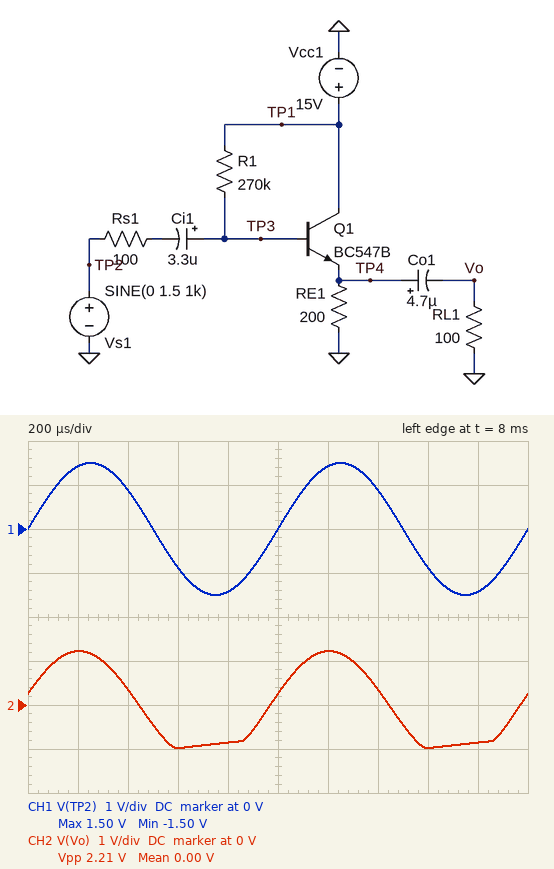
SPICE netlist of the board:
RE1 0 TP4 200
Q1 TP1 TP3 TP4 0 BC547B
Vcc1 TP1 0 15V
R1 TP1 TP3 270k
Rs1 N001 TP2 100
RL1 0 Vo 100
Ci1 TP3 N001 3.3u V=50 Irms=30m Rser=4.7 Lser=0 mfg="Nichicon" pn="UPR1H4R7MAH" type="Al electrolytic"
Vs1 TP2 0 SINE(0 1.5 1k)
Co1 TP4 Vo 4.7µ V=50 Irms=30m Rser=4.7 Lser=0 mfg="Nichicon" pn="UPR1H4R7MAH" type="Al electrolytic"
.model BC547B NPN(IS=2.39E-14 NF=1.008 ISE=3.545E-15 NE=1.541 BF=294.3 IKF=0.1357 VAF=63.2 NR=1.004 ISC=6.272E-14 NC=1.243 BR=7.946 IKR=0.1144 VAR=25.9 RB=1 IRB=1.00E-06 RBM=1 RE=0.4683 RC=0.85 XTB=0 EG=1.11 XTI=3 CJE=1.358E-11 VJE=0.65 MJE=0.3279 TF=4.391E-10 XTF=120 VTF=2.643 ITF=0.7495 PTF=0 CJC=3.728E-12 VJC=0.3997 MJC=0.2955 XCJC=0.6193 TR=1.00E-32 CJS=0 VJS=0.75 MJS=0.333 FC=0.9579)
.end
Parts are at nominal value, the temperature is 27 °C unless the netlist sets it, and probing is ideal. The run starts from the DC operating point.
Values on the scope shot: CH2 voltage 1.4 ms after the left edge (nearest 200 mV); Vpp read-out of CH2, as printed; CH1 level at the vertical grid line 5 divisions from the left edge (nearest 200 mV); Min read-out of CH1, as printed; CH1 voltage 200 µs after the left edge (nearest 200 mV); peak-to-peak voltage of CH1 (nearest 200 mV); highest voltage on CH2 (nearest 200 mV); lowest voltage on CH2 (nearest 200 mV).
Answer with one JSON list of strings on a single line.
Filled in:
["400 mV", "2.21 V", "0 V", "-1.50 V", "1.4 V", "3.0 V", "1.2 V", "-1.0 V"]
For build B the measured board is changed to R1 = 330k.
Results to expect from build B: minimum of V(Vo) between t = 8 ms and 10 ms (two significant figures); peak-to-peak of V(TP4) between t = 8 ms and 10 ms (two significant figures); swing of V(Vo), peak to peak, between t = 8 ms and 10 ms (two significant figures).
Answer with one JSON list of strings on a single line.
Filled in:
["-880 mV", "2.3 V", "2.1 V"]
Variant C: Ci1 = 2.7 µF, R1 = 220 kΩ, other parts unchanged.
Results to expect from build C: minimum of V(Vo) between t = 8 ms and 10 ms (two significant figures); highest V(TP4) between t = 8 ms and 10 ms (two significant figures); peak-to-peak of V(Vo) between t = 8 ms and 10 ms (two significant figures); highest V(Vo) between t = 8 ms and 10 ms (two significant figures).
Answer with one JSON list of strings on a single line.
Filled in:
["-1.1 V", "4.6 V", "2.4 V", "1.3 V"]
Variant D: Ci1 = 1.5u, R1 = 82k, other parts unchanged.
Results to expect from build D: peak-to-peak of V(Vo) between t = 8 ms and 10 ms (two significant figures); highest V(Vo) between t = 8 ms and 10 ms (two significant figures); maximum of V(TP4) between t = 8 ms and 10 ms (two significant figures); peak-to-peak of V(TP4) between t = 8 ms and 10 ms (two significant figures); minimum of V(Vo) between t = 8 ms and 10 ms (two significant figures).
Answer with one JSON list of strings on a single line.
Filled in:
["2.6 V", "1.3 V", "7.1 V", "2.9 V", "-1.3 V"]
